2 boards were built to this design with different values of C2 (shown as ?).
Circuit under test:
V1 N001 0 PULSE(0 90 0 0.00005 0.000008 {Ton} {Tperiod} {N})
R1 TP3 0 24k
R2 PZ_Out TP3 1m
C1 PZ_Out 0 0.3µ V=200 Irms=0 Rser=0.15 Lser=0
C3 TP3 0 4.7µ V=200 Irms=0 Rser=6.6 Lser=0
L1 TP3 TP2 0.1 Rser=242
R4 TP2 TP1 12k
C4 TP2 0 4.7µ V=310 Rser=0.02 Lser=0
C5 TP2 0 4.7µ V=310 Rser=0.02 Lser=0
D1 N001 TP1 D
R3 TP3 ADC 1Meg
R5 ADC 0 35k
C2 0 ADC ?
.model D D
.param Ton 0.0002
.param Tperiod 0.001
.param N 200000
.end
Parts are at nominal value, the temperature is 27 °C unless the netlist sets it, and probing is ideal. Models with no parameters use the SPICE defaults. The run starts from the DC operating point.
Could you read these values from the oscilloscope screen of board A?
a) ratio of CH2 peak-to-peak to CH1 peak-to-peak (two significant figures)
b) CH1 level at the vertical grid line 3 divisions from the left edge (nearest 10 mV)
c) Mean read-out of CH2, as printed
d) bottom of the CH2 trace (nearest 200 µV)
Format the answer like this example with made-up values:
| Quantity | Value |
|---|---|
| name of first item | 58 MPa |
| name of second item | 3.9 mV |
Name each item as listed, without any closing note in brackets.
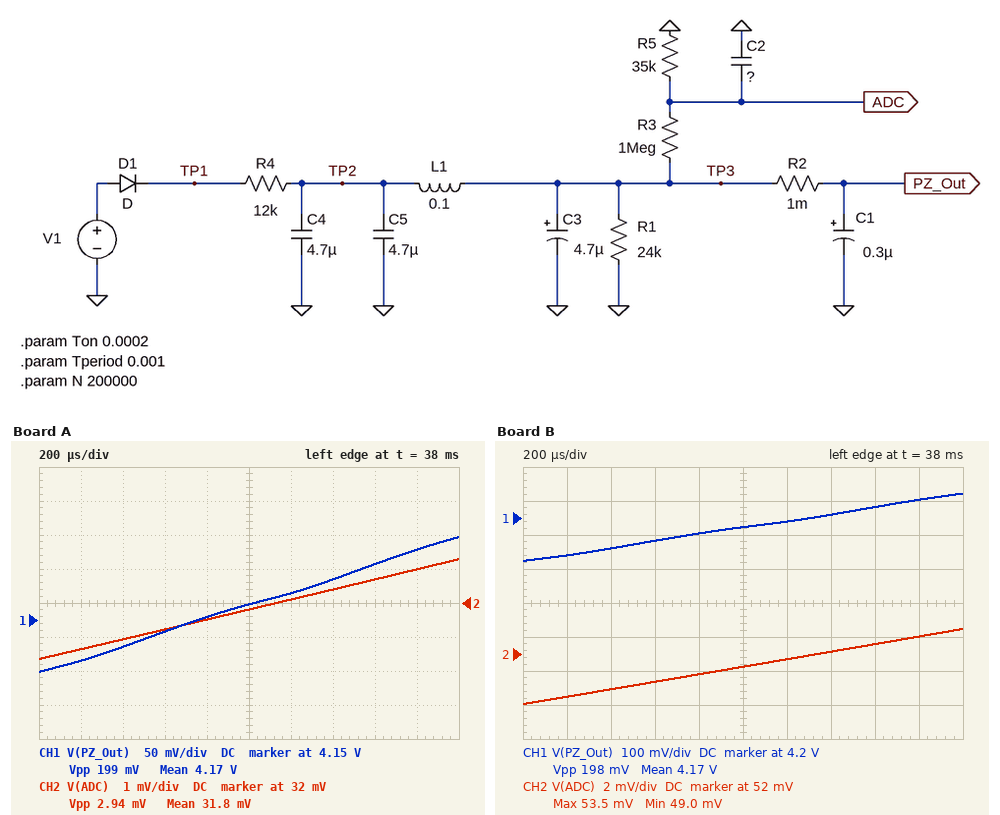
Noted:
| Quantity | Value |
|---|---|
| ratio of CH2 peak-to-peak to CH1 peak-to-peak | 0.015 |
| CH1 level at the vertical grid line 3 divisions from the left edge | 4.13 V |
| Mean read-out of CH2, as printed | 31.8 mV |
| bottom of the CH2 trace | 30.4 mV |
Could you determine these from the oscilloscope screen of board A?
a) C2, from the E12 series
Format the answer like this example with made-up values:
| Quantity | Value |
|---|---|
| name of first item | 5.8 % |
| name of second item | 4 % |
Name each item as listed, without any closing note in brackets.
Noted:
| Quantity | Value |
|---|---|
| C2, from the E12 series | 2.2 µF |
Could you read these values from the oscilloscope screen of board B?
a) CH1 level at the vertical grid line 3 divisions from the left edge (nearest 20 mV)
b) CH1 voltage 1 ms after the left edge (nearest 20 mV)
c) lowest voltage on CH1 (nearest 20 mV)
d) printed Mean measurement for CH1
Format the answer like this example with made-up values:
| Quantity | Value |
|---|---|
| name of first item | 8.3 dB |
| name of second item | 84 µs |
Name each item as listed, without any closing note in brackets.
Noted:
| Quantity | Value |
|---|---|
| CH1 level at the vertical grid line 3 divisions from the left edge | 4.14 V |
| CH1 voltage 1 ms after the left edge | 4.18 V |
| lowest voltage on CH1 | 4.08 V |
| printed Mean measurement for CH1 | 4.17 V |
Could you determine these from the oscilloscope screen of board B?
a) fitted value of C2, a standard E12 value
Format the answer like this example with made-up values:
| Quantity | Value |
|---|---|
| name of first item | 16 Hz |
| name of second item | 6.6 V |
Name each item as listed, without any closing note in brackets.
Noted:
| Quantity | Value |
|---|---|
| fitted value of C2, a standard E12 value | 1.2 µF |
